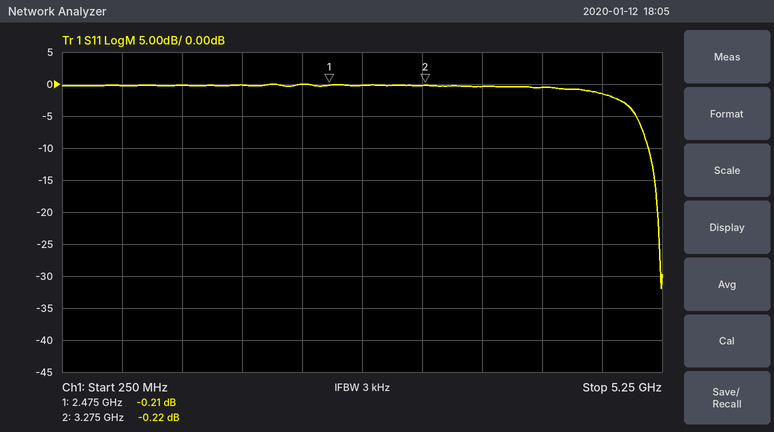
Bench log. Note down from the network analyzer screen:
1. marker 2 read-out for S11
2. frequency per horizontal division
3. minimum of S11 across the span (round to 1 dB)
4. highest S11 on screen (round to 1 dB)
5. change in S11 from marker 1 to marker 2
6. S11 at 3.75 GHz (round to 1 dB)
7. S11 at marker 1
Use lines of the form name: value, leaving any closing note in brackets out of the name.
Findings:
marker 2 read-out for S11: -0.22 dB
frequency per horizontal division: 500 MHz
minimum of S11 across the span: -32 dB
highest S11 on screen: 0 dB
change in S11 from marker 1 to marker 2: -0.01 dB
S11 at 3.75 GHz: 0 dB
S11 at marker 1: -0.21 dB
